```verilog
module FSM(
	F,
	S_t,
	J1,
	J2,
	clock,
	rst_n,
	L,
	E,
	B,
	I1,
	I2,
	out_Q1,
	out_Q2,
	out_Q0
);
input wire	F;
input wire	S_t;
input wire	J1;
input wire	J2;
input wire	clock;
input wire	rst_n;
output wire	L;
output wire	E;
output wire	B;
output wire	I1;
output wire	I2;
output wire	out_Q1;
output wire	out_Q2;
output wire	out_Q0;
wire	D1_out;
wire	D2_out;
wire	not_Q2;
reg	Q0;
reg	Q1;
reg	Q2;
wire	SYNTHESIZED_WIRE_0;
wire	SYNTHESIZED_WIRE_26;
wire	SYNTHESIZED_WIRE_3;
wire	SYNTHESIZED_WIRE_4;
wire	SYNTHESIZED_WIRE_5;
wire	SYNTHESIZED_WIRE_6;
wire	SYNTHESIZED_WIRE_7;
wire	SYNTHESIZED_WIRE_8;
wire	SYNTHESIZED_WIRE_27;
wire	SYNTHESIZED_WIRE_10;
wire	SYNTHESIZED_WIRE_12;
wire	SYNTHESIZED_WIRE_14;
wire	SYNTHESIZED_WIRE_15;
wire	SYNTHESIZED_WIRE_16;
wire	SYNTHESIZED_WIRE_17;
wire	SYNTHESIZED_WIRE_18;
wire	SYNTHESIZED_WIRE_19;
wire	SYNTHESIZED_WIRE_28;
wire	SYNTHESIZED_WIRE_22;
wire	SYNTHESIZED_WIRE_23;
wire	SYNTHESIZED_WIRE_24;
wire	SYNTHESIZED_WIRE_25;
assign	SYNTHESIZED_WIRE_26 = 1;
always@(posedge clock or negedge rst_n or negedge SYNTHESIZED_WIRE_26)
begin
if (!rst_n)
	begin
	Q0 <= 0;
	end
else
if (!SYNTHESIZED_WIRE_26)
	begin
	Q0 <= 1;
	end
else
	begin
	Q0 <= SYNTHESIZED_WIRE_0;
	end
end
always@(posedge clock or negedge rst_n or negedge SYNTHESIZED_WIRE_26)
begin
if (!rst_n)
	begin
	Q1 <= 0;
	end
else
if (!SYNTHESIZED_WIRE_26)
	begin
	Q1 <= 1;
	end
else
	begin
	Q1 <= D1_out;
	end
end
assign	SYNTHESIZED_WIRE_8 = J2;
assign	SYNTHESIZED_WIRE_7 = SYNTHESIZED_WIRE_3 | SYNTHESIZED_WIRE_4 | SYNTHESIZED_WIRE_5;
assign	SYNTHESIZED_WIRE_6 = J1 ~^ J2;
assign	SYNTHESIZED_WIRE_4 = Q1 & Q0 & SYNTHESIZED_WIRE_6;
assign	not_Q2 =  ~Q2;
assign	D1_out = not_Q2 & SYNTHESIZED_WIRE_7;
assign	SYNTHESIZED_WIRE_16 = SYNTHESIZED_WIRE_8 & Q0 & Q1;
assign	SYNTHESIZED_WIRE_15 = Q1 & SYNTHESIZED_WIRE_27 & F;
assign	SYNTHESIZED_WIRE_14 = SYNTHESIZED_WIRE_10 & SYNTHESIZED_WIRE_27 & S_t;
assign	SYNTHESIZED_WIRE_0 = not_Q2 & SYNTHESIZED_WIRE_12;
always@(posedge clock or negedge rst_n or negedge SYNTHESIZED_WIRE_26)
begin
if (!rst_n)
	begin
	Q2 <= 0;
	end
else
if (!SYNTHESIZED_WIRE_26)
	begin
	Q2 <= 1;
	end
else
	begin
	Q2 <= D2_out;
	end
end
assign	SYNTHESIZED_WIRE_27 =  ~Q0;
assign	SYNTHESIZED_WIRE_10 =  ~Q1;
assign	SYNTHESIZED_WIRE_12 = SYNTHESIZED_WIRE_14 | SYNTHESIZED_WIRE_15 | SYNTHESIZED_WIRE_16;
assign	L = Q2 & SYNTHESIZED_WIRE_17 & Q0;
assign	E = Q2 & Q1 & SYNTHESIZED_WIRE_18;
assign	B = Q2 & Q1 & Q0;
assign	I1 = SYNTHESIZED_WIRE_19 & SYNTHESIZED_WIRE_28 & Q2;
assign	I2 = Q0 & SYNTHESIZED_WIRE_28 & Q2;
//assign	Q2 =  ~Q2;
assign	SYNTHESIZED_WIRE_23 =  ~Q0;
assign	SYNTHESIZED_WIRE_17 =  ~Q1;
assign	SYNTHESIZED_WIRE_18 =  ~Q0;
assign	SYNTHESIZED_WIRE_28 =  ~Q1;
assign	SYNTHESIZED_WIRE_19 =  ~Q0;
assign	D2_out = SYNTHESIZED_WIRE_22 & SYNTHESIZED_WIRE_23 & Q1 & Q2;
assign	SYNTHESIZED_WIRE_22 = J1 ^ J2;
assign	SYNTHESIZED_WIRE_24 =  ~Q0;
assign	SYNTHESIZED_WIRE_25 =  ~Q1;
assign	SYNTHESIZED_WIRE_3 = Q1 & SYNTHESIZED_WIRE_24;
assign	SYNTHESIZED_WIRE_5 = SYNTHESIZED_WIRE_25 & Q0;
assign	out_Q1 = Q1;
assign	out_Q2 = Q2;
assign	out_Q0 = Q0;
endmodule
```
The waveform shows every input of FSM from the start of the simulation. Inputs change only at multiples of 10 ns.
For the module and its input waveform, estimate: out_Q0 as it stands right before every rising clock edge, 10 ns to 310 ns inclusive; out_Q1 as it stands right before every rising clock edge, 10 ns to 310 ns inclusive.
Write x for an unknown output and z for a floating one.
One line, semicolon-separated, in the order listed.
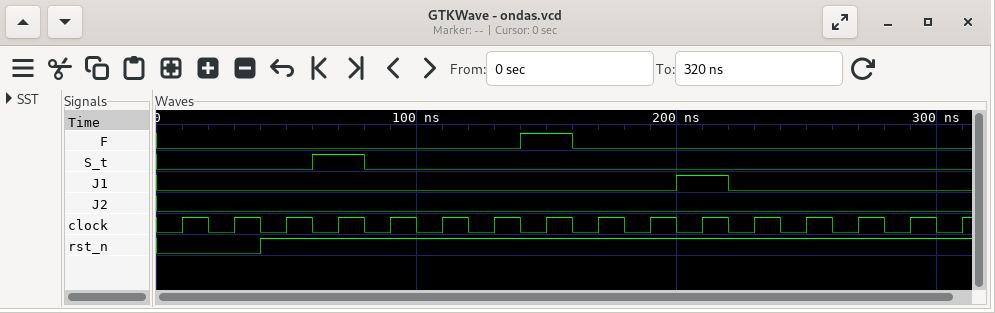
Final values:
0 0 0 0 1 0 0 0 1 0 0 0 0 0 0 0; 0 0 0 0 0 1 1 1 1 1 1 1 1 1 1 1
